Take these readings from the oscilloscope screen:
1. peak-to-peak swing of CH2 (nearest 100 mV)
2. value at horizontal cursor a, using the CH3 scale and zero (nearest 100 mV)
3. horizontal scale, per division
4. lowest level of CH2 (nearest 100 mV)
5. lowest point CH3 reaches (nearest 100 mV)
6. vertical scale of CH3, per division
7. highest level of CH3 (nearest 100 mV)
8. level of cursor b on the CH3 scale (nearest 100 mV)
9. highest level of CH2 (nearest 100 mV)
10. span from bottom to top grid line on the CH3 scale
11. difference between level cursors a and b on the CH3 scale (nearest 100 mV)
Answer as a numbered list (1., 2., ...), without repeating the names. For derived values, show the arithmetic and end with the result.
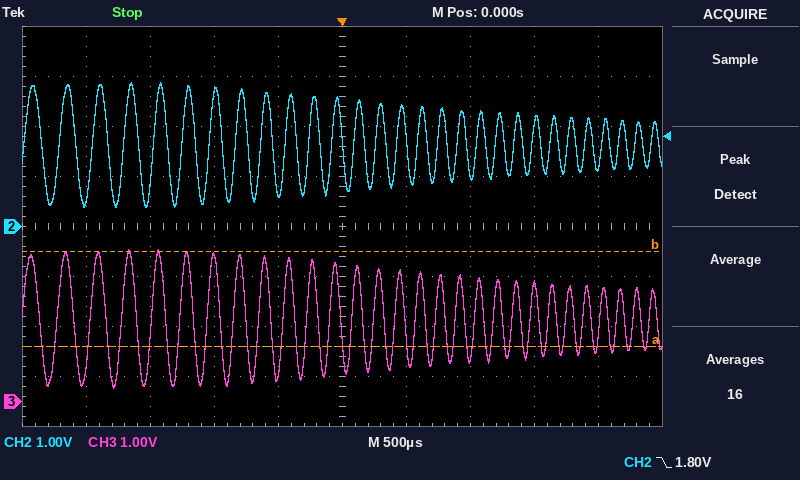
1. 2.9 V − (400 mV) = 2.5 V
2. 1.1 V
3. 500 µs
4. 400 mV
5. 300 mV
6. 1 V
7. 3.0 V
8. 3.0 V
9. 2.9 V
10. 8 V
11. 1.9 V
